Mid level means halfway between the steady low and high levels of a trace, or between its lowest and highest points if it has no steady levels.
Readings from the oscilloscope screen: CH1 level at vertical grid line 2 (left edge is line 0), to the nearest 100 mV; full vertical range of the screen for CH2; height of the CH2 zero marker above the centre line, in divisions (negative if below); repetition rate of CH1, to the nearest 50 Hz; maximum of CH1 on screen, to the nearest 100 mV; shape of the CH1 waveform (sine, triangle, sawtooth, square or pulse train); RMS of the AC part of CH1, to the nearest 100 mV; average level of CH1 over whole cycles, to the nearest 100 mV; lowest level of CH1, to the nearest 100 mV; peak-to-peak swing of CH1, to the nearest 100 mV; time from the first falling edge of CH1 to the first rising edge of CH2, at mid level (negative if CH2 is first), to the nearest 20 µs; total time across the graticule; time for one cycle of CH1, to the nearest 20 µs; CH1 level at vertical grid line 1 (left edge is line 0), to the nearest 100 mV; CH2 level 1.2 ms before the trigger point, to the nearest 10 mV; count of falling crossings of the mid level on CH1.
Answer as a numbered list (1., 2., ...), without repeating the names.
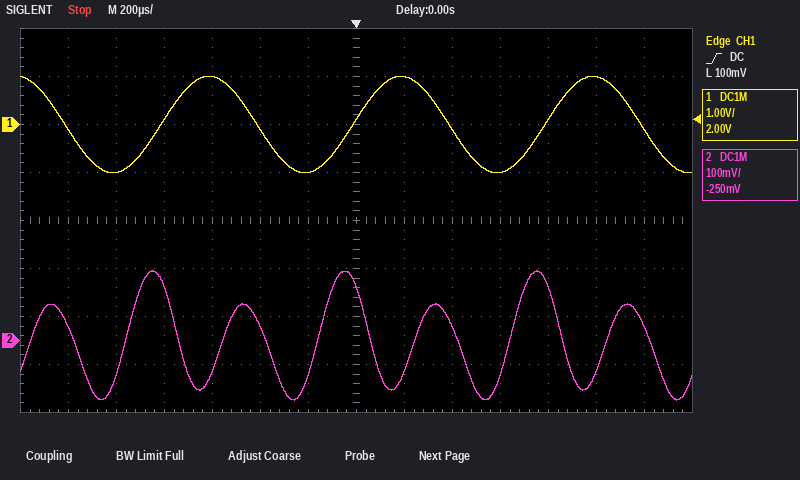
1. -1.0 V
2. 800 mV
3. -2.5 div
4. 1.25 kHz
5. 1.0 V
6. sine
7. 700 mV
8. 0.0 V
9. -1.0 V
10. 2.0 V
11. -140 µs
12. 2.8 ms
13. 800 µs
14. -100 mV
15. 30 mV
16. 4
